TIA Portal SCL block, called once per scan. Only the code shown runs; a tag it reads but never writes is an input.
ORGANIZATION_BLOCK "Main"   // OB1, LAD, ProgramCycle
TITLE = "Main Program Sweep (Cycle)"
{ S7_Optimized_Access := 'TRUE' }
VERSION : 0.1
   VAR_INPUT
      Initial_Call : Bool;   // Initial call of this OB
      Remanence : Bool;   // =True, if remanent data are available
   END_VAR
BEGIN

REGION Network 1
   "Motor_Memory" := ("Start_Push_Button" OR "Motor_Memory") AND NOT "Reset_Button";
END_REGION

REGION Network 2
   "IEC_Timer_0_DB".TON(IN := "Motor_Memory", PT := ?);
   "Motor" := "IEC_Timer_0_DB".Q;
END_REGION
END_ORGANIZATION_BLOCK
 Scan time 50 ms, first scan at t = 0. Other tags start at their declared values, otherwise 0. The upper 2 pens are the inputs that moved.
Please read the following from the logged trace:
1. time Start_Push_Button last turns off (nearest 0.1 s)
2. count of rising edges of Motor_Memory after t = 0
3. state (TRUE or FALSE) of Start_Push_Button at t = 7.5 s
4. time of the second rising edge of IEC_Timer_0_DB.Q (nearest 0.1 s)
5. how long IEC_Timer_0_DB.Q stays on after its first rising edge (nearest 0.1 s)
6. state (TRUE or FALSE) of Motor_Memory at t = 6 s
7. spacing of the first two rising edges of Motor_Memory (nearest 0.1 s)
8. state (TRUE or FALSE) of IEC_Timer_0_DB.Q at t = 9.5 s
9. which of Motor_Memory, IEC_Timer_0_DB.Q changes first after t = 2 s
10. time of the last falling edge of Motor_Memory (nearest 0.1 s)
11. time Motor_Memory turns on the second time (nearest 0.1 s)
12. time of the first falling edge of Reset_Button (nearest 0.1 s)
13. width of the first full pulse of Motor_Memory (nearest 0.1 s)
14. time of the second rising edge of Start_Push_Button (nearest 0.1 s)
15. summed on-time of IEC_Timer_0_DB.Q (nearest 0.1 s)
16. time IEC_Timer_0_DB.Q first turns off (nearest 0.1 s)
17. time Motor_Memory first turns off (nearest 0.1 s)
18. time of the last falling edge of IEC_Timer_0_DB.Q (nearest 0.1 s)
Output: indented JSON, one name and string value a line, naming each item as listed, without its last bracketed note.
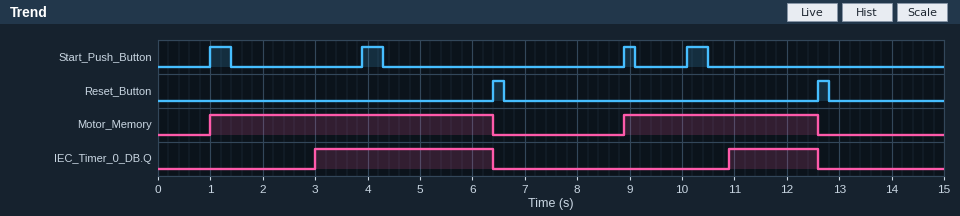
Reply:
{
  "time Start_Push_Button last turns off": "10.5 s",
  "count of rising edges of Motor_Memory after t = 0": "2",
  "state (TRUE or FALSE) of Start_Push_Button at t = 7.5 s": "FALSE",
  "time of the second rising edge of IEC_Timer_0_DB.Q": "10.9 s",
  "how long IEC_Timer_0_DB.Q stays on after its first rising edge": "3.4 s",
  "state (TRUE or FALSE) of Motor_Memory at t = 6 s": "TRUE",
  "spacing of the first two rising edges of Motor_Memory": "7.9 s",
  "state (TRUE or FALSE) of IEC_Timer_0_DB.Q at t = 9.5 s": "FALSE",
  "which of Motor_Memory, IEC_Timer_0_DB.Q changes first after t = 2 s": "IEC_Timer_0_DB.Q",
  "time of the last falling edge of Motor_Memory": "12.6 s",
  "time Motor_Memory turns on the second time": "8.9 s",
  "time of the first falling edge of Reset_Button": "6.6 s",
  "width of the first full pulse of Motor_Memory": "5.4 s",
  "time of the second rising edge of Start_Push_Button": "3.9 s",
  "summed on-time of IEC_Timer_0_DB.Q": "5.1 s",
  "time IEC_Timer_0_DB.Q first turns off": "6.4 s",
  "time Motor_Memory first turns off": "6.4 s",
  "time of the last falling edge of IEC_Timer_0_DB.Q": "12.6 s"
}
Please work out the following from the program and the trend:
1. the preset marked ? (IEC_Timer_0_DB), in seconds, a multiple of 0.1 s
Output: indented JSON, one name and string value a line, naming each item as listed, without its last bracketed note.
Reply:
{
  "the preset marked ? (IEC_Timer_0_DB), in seconds, a multiple of 0.1 s": "2.0 s"
}
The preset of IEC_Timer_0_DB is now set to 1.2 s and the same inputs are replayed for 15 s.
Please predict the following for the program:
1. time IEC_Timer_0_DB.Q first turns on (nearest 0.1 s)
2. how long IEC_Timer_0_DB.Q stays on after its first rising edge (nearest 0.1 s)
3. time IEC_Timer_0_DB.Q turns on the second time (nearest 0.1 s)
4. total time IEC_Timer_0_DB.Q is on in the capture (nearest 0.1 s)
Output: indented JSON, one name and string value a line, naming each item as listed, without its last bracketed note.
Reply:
{
  "time IEC_Timer_0_DB.Q first turns on": "2.2 s",
  "how long IEC_Timer_0_DB.Q stays on after its first rising edge": "4.2 s",
  "time IEC_Timer_0_DB.Q turns on the second time": "10.1 s",
  "total time IEC_Timer_0_DB.Q is on in the capture": "6.7 s"
}
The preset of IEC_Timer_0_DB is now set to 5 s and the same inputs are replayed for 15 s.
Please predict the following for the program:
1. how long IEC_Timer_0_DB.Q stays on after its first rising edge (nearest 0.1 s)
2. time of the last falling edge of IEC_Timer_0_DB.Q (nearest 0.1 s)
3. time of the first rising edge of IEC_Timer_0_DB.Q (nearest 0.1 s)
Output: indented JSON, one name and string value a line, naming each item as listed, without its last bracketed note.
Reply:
{
  "how long IEC_Timer_0_DB.Q stays on after its first rising edge": "0.4 s",
  "time of the last falling edge of IEC_Timer_0_DB.Q": "6.4 s",
  "time of the first rising edge of IEC_Timer_0_DB.Q": "6.0 s"
}
